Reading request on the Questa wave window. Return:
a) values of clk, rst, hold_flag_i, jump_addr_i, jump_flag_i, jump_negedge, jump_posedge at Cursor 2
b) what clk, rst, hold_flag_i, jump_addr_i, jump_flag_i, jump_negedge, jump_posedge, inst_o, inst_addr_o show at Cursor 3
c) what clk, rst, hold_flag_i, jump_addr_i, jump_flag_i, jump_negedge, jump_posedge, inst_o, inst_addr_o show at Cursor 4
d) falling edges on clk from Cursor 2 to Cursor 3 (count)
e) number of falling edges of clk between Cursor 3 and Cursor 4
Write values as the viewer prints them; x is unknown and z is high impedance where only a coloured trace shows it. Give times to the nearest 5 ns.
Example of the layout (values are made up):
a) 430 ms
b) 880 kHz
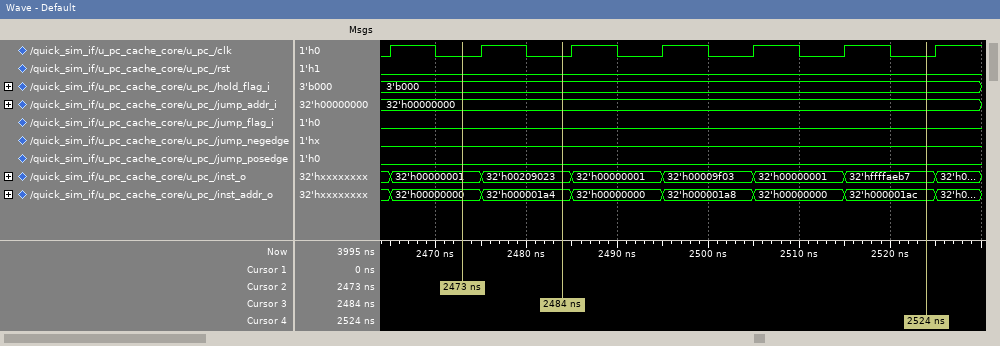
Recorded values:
a) clk=0, rst=0, hold_flag_i=3'b000, jump_addr_i=32'h00000000, jump_flag_i=0, jump_negedge=0, jump_posedge=0
b) clk=0, rst=0, hold_flag_i=3'b000, jump_addr_i=32'h00000000, jump_flag_i=0, jump_negedge=0, jump_posedge=0, inst_o=32'h00209023, inst_addr_o=32'h000001a4
c) clk=0, rst=0, hold_flag_i=3'b000, jump_addr_i=32'h00000000, jump_flag_i=0, jump_negedge=0, jump_posedge=0, inst_o=32'hffffaeb7, inst_addr_o=32'h000001ac
d) 1
e) 4
